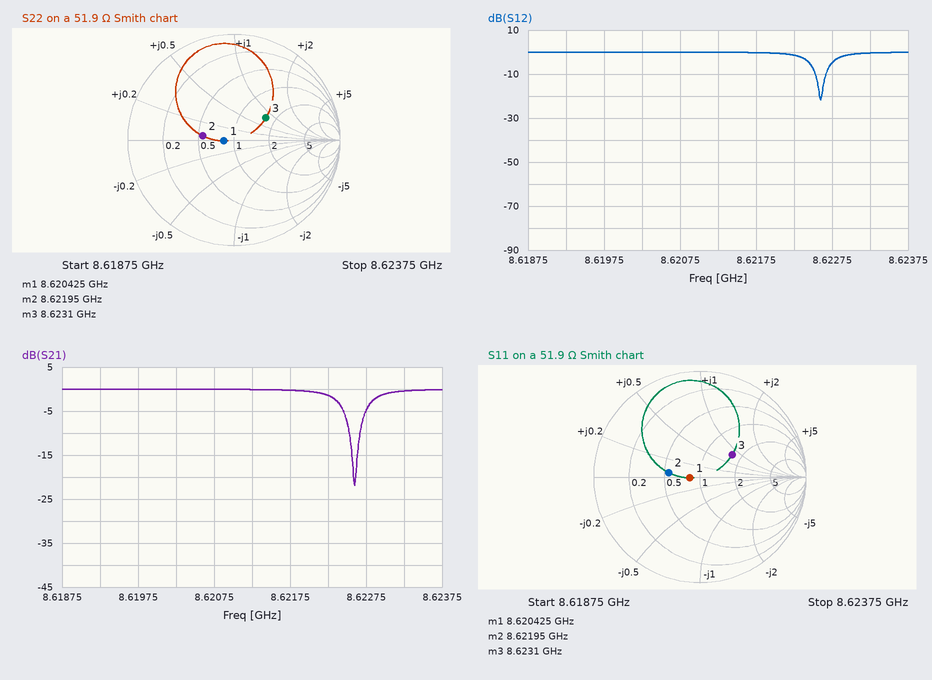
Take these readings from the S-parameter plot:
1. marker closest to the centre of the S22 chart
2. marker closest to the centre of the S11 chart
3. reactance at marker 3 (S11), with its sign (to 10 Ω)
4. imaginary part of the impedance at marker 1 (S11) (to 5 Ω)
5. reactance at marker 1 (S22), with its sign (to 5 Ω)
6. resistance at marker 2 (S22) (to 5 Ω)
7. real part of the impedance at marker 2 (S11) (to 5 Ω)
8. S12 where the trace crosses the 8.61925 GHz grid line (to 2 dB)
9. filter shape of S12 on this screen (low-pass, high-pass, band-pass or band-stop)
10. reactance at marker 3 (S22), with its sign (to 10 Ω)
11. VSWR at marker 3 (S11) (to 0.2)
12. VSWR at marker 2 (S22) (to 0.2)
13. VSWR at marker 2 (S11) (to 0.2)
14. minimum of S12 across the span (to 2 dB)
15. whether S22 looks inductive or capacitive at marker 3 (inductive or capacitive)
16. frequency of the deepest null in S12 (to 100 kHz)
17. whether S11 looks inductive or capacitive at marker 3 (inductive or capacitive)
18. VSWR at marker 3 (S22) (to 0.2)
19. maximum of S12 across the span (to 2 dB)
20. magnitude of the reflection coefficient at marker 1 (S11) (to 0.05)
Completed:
marker 1
marker 1
+40 Ω
0 Ω
0 Ω
30 Ω
30 Ω
0 dB
band-stop
+40 Ω
2.2
1.8
1.8
-22 dB
inductive
8.6226 GHz
inductive
2.2
0 dB
0.10
